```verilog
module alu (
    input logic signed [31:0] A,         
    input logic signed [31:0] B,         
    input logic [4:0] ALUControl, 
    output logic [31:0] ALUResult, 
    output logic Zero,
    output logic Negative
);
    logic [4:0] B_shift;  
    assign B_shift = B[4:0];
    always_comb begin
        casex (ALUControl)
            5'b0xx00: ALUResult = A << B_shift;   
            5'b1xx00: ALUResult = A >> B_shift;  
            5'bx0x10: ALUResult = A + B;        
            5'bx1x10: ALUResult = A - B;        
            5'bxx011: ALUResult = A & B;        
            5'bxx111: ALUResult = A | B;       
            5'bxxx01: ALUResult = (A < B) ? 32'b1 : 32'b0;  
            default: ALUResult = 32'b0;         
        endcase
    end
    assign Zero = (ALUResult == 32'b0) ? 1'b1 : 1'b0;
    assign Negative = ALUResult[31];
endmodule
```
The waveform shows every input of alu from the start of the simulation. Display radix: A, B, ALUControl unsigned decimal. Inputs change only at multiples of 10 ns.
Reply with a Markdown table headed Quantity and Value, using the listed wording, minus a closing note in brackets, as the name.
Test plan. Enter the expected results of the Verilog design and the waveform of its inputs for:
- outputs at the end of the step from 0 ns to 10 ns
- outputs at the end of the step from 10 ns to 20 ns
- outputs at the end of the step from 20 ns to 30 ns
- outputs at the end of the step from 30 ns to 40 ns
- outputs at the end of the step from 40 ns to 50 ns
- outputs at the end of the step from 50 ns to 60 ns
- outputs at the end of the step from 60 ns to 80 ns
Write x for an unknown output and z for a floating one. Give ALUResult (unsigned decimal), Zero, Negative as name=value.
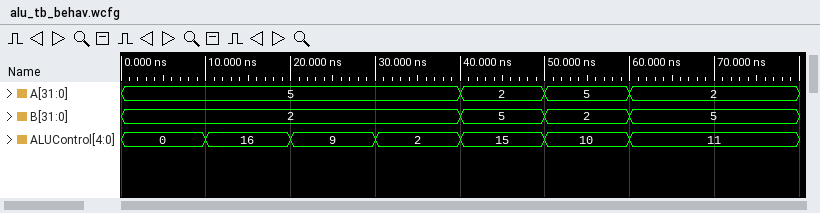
| Quantity | Value |
|---|---|
| outputs at the end of the step from 0 ns to 10 ns | ALUResult=20, Zero=0, Negative=0 |
| outputs at the end of the step from 10 ns to 20 ns | ALUResult=1, Zero=0, Negative=0 |
| outputs at the end of the step from 20 ns to 30 ns | ALUResult=0, Zero=1, Negative=0 |
| outputs at the end of the step from 30 ns to 40 ns | ALUResult=7, Zero=0, Negative=0 |
| outputs at the end of the step from 40 ns to 50 ns | ALUResult=7, Zero=0, Negative=0 |
| outputs at the end of the step from 50 ns to 60 ns | ALUResult=3, Zero=0, Negative=0 |
| outputs at the end of the step from 60 ns to 80 ns | ALUResult=0, Zero=1, Negative=0 |
